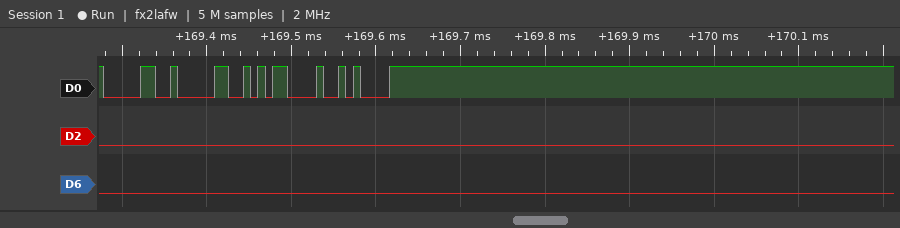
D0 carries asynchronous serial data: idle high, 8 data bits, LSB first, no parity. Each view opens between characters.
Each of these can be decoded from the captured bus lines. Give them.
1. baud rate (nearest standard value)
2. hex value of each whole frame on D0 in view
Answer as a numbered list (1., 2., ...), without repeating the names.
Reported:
1. 115200 baud
2. 30, 30, 0D, 0A
